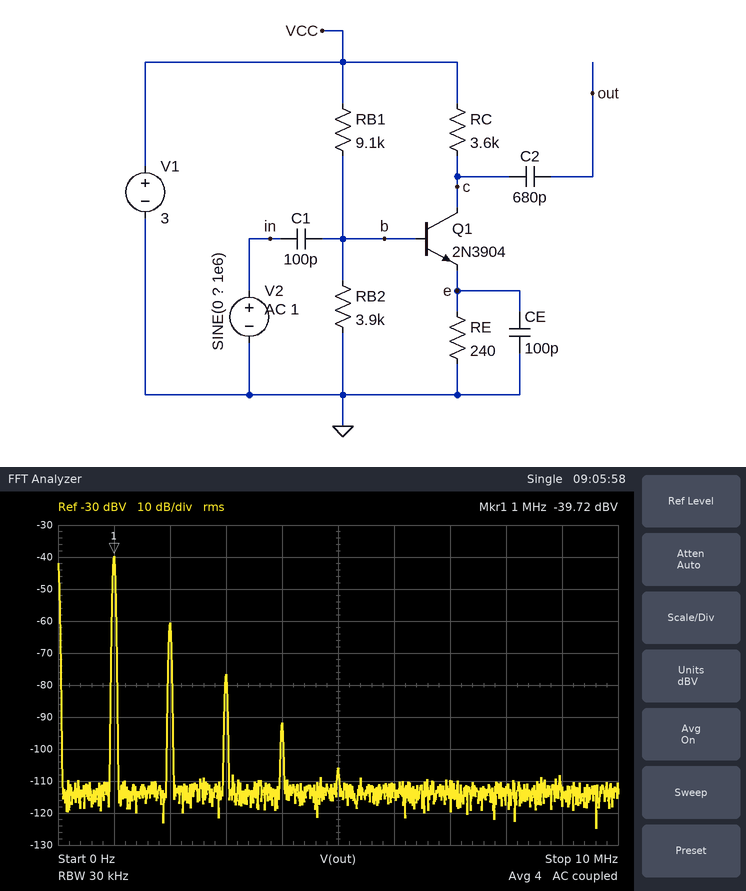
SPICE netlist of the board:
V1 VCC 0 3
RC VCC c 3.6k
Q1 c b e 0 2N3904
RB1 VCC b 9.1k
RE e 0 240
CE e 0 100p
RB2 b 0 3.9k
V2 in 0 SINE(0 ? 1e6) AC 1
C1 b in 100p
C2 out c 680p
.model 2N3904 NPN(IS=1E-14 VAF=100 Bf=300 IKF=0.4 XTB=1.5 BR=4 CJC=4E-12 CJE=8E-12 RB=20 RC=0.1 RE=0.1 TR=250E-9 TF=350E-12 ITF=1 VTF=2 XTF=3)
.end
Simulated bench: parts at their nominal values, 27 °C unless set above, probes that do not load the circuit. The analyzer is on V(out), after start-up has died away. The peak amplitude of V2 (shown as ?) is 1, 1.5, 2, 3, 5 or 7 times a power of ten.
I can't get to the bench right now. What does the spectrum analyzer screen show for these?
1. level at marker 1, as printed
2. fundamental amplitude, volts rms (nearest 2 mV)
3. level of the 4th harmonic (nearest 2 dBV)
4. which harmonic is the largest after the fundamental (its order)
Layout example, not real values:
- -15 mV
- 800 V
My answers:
- -39.72 dBV
- 10 mV
- -92 dBV
- 2
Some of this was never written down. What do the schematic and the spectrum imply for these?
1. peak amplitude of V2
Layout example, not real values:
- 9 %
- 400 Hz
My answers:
- 100 mV
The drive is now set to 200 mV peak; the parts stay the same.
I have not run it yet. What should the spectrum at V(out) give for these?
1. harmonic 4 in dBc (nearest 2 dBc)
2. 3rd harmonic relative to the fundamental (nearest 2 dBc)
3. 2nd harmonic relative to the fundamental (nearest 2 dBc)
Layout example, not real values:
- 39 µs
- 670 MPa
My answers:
- -28 dBc
- -20 dBc
- -12 dBc
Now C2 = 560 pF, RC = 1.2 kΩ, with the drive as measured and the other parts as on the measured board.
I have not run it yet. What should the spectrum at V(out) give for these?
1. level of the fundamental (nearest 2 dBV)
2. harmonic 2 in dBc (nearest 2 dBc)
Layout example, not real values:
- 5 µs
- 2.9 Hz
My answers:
- -12 dBV
- -48 dBc
